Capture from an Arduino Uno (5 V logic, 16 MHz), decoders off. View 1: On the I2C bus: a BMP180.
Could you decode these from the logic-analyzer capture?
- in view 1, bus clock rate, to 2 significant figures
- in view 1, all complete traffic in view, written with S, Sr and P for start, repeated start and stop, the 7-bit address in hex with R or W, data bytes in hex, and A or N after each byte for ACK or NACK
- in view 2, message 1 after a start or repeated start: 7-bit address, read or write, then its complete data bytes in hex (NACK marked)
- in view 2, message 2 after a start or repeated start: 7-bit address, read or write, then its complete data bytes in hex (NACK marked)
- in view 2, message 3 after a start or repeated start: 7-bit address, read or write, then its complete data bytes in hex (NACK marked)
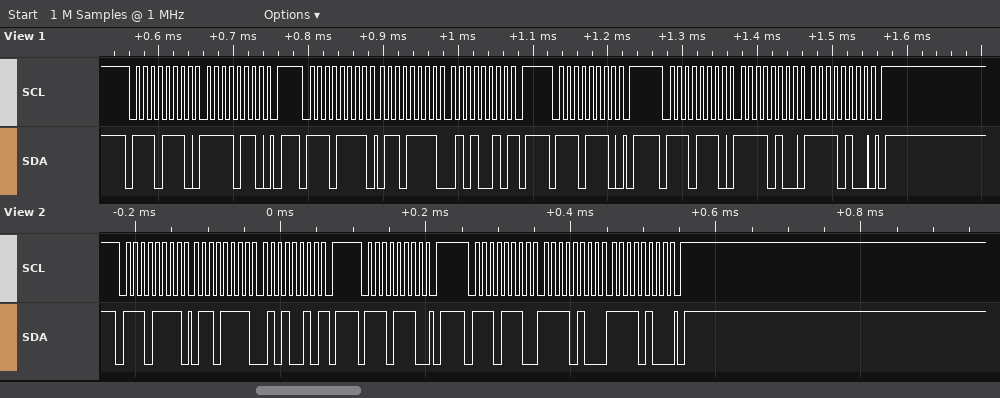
100 kHz
S 77W A F6 A P S 77R A 6F A 52 N P S 77W A P S 77W A F4 A F4 A P
0x77 read: 6F 52 NACK
0x77 write
0x77 write: F4 F4
